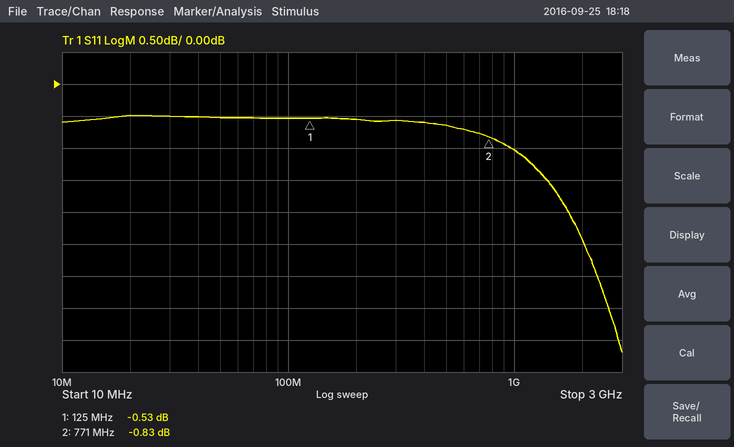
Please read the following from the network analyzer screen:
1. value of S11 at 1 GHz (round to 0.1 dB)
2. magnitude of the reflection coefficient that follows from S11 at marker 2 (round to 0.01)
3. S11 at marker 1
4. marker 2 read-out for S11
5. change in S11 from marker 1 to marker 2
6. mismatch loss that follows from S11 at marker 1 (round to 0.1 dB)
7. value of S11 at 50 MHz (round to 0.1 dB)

-1.0 dB
0.91
-0.53 dB
-0.83 dB
-0.30 dB
9.4 dB
-0.5 dB
